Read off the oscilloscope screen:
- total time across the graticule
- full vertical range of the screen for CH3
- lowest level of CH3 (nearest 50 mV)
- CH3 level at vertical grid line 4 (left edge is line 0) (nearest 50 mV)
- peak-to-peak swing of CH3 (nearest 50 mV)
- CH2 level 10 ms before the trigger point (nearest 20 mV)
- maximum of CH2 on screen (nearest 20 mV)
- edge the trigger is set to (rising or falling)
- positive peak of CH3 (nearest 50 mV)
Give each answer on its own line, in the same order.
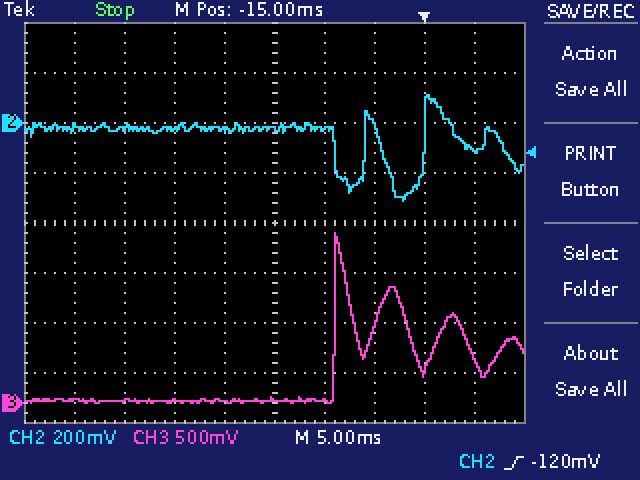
50 ms
4 V
0 mV
0 mV
1.70 V
-20 mV
120 mV
rising
1.70 V
